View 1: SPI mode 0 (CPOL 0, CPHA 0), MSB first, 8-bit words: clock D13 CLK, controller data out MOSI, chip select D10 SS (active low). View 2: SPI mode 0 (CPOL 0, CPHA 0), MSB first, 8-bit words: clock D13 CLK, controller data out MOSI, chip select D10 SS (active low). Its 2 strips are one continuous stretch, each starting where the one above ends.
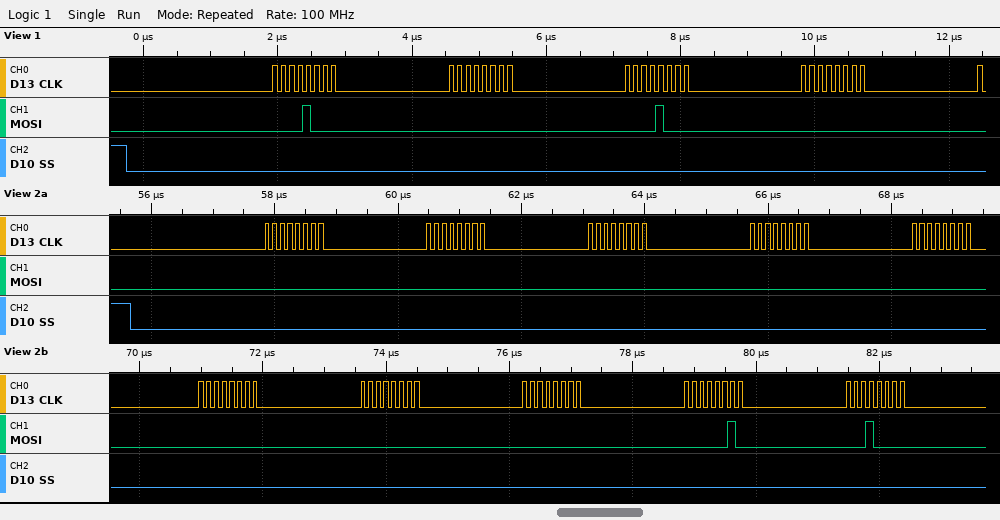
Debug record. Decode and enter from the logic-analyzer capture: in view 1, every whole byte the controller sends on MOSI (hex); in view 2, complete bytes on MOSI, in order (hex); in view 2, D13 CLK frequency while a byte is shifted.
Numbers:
08 00 08 00
00 00 00 00 00 00 00 00 02 10
8 MHz
